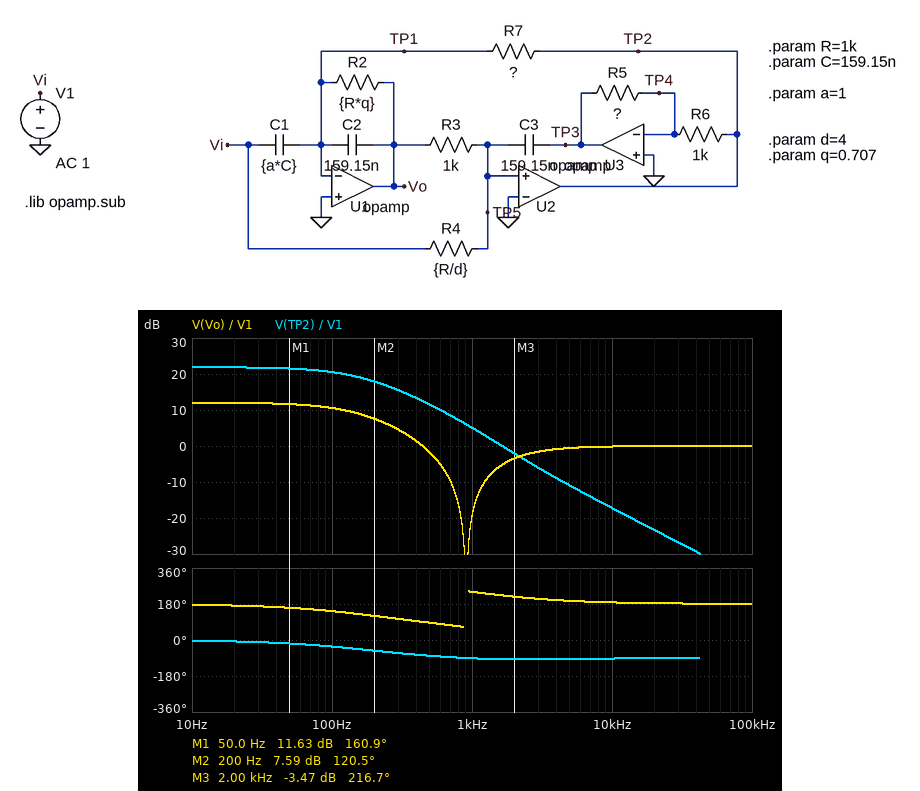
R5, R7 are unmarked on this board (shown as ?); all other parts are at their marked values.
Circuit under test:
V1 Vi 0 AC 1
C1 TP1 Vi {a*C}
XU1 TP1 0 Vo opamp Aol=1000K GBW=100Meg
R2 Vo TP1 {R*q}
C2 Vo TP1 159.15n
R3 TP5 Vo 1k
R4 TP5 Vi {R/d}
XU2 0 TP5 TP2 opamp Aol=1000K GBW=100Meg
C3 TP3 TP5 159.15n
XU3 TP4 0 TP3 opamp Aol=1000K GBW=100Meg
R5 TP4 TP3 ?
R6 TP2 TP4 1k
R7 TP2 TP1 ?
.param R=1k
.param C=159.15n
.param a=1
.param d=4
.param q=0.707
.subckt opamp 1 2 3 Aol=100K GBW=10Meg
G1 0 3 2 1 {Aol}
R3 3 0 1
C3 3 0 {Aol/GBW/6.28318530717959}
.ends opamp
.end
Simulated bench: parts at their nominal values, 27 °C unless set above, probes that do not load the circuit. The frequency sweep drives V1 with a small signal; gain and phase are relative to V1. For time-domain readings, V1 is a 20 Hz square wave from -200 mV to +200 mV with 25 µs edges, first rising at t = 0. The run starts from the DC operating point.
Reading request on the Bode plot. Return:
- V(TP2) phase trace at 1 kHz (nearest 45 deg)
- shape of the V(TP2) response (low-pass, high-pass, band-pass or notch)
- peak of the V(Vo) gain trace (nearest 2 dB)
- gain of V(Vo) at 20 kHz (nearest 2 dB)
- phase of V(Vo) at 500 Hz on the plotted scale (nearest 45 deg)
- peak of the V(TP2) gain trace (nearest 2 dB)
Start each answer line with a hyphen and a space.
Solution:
- -90 deg
- low-pass
- 12 dB
- 0 dB
- 90 deg
- 22 dB
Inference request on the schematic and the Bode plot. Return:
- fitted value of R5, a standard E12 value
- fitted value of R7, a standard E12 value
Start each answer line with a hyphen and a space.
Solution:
- 2.2 kΩ
- 2.2 kΩ
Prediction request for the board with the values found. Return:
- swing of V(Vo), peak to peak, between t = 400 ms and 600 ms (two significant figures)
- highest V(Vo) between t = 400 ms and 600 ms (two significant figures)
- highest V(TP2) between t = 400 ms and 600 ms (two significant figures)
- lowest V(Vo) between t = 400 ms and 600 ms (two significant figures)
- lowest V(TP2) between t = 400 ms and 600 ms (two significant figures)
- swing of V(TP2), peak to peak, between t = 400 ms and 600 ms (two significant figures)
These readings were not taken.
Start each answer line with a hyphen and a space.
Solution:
- 1.6 V
- 800 mV
- 2.5 V
- -800 mV
- -2.5 V
- 5.0 V
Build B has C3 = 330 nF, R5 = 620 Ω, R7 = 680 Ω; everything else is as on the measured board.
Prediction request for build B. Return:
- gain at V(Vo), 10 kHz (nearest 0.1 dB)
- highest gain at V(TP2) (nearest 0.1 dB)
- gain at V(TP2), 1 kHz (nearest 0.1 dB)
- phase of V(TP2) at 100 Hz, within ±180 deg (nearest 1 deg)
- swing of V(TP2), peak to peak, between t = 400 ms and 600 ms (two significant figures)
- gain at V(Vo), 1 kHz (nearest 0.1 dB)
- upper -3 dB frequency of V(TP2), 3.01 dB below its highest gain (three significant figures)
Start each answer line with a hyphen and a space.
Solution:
- -0.4 dB
- 12.0 dB
- 10.9 dB
- -4 deg
- 1.8 V
- 8.0 dB
- 1.28 kHz
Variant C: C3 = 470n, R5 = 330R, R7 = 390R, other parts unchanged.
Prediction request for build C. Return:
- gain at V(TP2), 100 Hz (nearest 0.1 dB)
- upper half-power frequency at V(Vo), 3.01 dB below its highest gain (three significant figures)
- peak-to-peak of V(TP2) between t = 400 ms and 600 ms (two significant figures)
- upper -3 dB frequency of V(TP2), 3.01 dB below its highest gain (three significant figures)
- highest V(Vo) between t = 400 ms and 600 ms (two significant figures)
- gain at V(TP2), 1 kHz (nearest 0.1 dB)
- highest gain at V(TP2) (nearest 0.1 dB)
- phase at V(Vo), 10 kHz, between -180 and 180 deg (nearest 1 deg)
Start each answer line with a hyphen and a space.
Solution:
- 6.9 dB
- 1.71 kHz
- 1.5 V
- 2.14 kHz
- 1.1 V
- 9.7 dB
- 10.8 dB
- -172 deg
